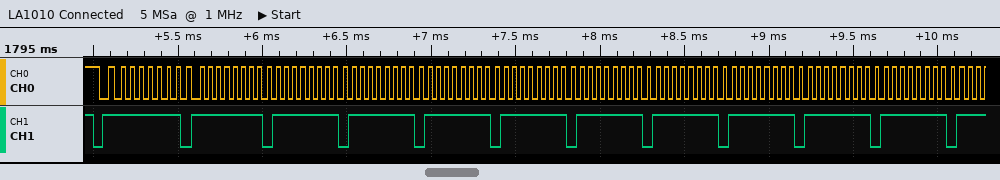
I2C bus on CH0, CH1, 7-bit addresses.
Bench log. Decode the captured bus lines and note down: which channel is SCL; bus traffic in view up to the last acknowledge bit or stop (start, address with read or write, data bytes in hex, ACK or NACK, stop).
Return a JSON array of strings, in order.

["CH0", "start, address 7F read ACK, FF ACK, FF ACK, FF ACK, FF ACK, FF ACK, FF ACK, FF ACK, FF ACK, FF ACK, FF ACK"]
